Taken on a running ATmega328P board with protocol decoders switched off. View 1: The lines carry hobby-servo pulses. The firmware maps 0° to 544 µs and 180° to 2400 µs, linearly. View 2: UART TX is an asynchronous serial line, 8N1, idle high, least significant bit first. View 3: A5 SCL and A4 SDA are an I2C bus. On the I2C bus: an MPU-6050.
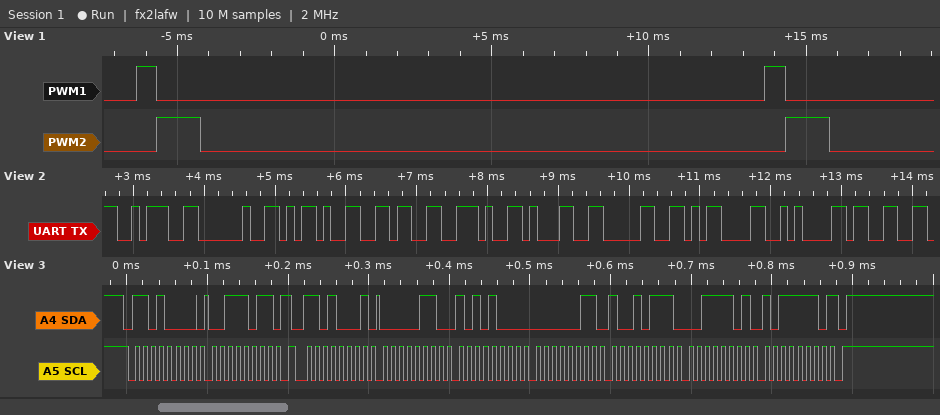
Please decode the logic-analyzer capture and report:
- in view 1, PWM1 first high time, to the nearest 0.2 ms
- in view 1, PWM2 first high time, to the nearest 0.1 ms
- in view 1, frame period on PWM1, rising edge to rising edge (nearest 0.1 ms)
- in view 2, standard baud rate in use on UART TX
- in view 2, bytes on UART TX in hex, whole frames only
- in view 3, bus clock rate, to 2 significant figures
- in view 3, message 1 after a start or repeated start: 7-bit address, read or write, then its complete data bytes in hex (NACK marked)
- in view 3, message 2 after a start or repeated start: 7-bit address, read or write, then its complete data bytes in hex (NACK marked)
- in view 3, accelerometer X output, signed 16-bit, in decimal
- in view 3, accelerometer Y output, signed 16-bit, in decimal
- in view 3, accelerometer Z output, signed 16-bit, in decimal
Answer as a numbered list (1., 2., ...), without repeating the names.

1. 0.6 ms
2. 1.4 ms
3. 20.0 ms
4. 9600 baud
5. 3A 20 2D 36 2E 31 30 0D 0A 33
6. 100 kHz
7. 0x68 write: 3B
8. 0x68 read: 06 A8 03 97 3D BE NACK
9. 1704
10. 919
11. 15806
